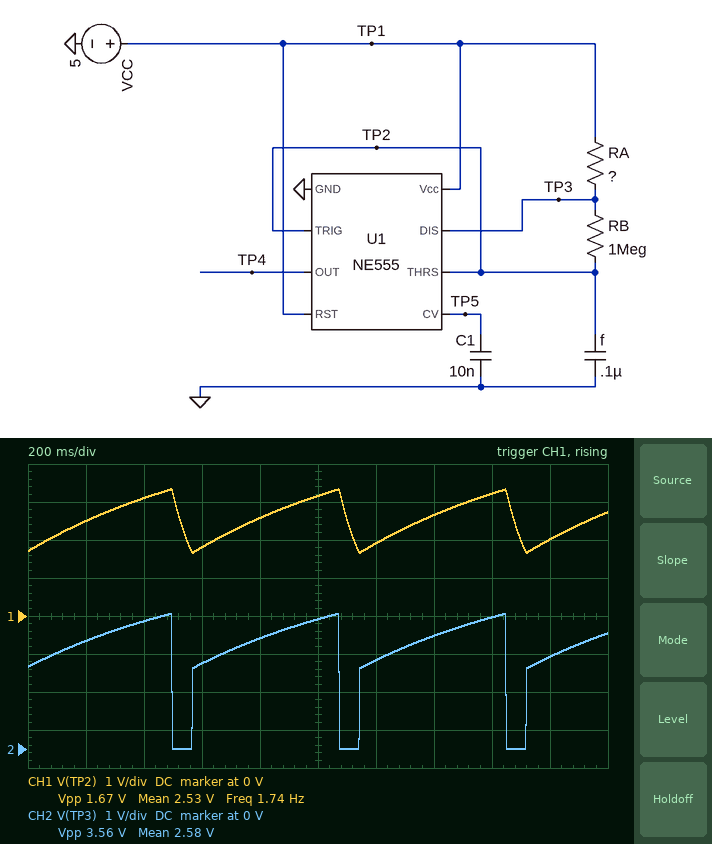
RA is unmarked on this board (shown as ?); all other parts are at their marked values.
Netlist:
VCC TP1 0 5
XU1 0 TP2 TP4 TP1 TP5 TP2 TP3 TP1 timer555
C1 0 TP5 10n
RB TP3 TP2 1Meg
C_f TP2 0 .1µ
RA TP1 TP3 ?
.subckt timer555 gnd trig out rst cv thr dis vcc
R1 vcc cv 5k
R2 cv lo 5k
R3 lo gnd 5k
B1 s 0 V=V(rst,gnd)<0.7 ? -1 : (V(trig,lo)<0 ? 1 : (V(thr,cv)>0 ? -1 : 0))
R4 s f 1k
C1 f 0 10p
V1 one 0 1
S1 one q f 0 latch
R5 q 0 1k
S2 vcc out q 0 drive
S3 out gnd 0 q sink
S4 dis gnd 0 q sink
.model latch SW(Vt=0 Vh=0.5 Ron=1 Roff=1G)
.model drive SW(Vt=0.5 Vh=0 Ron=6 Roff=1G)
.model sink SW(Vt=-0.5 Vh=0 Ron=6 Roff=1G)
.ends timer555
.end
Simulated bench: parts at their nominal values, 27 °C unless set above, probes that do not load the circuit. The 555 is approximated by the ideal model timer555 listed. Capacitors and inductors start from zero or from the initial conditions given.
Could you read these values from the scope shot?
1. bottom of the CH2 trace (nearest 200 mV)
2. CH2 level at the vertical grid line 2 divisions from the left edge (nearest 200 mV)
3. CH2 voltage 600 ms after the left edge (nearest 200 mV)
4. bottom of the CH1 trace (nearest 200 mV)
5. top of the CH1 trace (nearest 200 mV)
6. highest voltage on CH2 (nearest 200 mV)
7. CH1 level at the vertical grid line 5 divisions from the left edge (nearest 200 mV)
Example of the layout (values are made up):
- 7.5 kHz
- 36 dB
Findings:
- 0 V
- 3.4 V
- 2.2 V
- 1.6 V
- 3.4 V
- 3.6 V
- 3.2 V
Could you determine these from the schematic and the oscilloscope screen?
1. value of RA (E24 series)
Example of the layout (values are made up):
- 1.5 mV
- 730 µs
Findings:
- 6.2 MΩ
